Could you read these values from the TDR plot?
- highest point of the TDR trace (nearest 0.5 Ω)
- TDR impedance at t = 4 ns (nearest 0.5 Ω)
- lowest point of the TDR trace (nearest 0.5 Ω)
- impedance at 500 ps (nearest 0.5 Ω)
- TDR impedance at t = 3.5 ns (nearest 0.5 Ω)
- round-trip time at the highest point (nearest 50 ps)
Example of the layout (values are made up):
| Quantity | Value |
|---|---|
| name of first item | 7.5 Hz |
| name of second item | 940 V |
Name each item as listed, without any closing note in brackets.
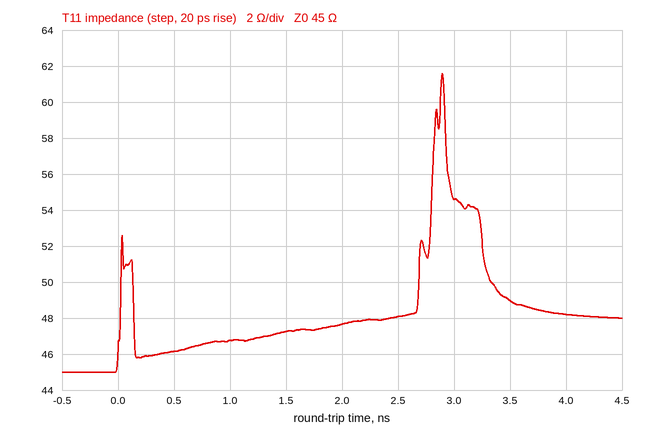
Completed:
| Quantity | Value |
|---|---|
| highest point of the TDR trace | 61.5 Ω |
| TDR impedance at t = 4 ns | 48.0 Ω |
| lowest point of the TDR trace | 45.0 Ω |
| impedance at 500 ps | 46.0 Ω |
| TDR impedance at t = 3.5 ns | 49.0 Ω |
| round-trip time at the highest point | 2.90 ns |
